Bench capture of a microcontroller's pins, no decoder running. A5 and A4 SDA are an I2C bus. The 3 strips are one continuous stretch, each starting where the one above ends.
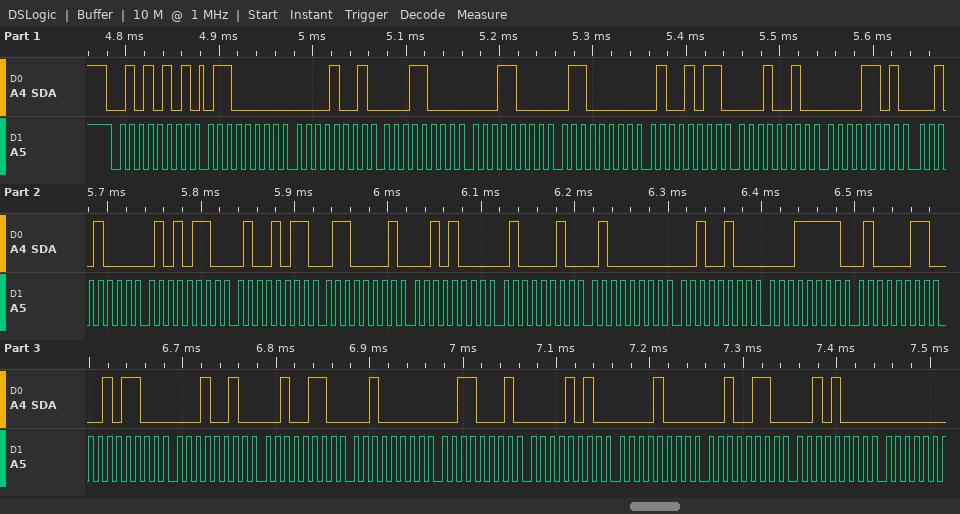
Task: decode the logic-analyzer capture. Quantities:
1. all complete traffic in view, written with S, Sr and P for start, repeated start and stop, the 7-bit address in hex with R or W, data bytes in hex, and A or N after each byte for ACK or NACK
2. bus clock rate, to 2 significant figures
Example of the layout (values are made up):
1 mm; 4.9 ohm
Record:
S 2AR A 60 A 09 A 18 A 18 A 60 A 4B A 12 A 0D A 28 A 56 A 4B A 61 A 28 A 42 A 40 A 24 A 1F A 43 A 2C A 12 A 26 A 20 A 31 A 0A A 08 A 26 A 28 A; 100 kHz
